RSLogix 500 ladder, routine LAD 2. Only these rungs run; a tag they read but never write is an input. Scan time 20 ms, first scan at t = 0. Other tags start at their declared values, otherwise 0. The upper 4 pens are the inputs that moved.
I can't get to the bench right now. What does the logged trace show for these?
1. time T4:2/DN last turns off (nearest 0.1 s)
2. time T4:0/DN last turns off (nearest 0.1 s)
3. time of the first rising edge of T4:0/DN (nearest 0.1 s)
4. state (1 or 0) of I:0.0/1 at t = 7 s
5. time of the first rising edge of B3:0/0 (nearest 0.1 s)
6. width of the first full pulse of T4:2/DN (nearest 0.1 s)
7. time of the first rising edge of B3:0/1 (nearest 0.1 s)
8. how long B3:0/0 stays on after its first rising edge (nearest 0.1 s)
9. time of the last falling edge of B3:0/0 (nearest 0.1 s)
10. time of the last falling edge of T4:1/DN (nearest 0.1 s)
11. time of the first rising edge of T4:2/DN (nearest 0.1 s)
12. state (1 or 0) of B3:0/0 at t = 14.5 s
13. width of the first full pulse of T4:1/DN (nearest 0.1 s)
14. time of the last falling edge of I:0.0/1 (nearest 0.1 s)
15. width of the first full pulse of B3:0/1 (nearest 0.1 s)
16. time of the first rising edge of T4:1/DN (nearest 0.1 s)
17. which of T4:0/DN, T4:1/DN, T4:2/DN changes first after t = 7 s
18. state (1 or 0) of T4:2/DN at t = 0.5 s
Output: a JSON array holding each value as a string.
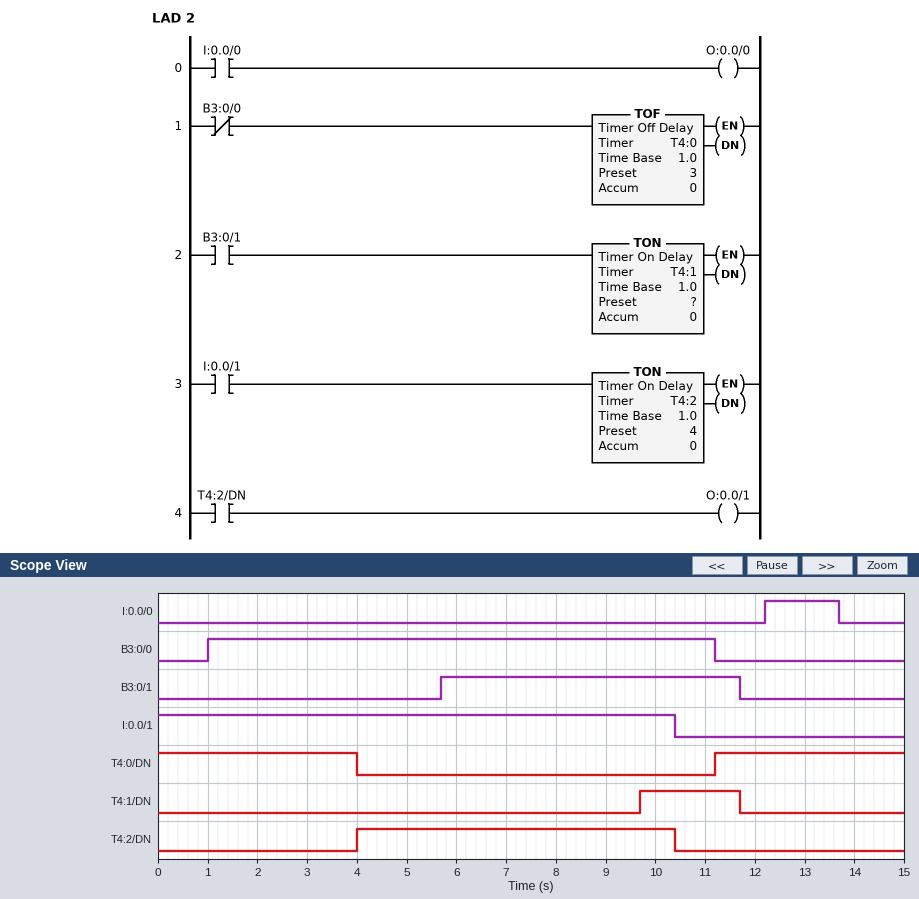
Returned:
["10.4 s", "4.0 s", "11.2 s", "1", "1.0 s", "6.4 s", "5.7 s", "10.2 s", "11.2 s", "11.7 s", "4.0 s", "0", "2.0 s", "10.4 s", "6.0 s", "9.7 s", "T4:1/DN", "0"]
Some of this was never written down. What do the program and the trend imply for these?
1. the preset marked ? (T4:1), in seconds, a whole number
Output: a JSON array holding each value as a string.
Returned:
["4 s"]
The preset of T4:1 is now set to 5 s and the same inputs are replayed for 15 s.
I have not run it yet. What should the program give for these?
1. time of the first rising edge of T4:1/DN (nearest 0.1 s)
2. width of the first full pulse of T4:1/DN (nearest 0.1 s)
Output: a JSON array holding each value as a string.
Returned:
["10.7 s", "1.0 s"]
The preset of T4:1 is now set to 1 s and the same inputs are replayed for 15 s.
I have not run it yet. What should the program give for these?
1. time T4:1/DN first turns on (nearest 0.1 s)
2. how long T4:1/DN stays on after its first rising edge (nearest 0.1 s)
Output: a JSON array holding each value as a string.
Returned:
["6.7 s", "5.0 s"]
